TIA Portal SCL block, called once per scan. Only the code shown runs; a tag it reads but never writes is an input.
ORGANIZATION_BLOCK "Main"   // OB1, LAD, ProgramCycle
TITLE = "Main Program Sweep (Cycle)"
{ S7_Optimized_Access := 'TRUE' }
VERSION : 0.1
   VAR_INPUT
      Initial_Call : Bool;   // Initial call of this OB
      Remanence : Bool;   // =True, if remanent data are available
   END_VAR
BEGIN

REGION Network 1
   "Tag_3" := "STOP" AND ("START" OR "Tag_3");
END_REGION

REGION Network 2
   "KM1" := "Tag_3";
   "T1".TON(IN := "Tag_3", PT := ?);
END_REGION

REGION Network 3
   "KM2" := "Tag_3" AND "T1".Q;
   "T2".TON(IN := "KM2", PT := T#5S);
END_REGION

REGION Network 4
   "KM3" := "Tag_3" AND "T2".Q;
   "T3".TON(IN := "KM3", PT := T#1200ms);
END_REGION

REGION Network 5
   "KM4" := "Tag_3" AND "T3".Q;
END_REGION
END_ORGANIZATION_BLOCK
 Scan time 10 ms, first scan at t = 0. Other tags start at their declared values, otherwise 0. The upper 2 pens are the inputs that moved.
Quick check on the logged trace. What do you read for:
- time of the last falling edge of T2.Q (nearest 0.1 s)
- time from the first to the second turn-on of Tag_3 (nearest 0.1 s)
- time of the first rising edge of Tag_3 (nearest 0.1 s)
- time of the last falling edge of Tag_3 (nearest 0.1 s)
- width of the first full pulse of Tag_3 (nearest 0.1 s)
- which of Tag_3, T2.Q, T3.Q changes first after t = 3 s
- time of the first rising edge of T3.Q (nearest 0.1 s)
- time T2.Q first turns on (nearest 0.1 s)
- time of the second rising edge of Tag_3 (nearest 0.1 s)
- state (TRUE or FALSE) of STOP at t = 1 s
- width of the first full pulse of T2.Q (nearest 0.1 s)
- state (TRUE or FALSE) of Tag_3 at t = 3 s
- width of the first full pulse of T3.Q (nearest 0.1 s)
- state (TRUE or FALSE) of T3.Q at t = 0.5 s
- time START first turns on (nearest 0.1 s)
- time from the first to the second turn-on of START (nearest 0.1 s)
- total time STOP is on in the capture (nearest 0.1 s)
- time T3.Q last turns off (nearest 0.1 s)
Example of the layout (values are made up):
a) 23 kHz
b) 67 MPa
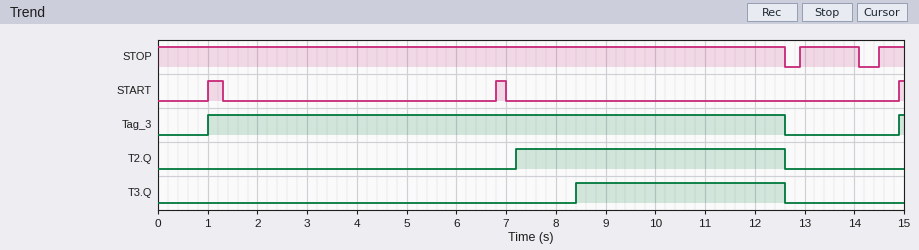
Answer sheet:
a) 12.6 s
b) 13.9 s
c) 1.0 s
d) 12.6 s
e) 11.6 s
f) T2.Q
g) 8.4 s
h) 7.2 s
i) 14.9 s
j) TRUE
k) 5.4 s
l) TRUE
m) 4.2 s
n) FALSE
o) 1.0 s
p) 5.8 s
q) 14.3 s
r) 12.6 s
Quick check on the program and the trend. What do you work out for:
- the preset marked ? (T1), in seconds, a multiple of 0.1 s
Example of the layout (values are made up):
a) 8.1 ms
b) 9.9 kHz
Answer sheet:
a) 1.2 s
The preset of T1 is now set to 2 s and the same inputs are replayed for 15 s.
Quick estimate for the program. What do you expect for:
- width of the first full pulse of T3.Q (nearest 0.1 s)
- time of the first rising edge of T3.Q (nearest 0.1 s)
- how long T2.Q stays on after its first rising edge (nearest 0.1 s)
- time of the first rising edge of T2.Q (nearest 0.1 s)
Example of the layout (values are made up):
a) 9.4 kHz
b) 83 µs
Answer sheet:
a) 3.4 s
b) 9.2 s
c) 4.6 s
d) 8.0 s
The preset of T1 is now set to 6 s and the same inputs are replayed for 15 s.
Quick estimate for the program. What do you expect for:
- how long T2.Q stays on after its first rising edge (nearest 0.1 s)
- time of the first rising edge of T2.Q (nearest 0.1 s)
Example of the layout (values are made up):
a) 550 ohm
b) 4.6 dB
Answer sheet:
a) 0.6 s
b) 12.0 s
